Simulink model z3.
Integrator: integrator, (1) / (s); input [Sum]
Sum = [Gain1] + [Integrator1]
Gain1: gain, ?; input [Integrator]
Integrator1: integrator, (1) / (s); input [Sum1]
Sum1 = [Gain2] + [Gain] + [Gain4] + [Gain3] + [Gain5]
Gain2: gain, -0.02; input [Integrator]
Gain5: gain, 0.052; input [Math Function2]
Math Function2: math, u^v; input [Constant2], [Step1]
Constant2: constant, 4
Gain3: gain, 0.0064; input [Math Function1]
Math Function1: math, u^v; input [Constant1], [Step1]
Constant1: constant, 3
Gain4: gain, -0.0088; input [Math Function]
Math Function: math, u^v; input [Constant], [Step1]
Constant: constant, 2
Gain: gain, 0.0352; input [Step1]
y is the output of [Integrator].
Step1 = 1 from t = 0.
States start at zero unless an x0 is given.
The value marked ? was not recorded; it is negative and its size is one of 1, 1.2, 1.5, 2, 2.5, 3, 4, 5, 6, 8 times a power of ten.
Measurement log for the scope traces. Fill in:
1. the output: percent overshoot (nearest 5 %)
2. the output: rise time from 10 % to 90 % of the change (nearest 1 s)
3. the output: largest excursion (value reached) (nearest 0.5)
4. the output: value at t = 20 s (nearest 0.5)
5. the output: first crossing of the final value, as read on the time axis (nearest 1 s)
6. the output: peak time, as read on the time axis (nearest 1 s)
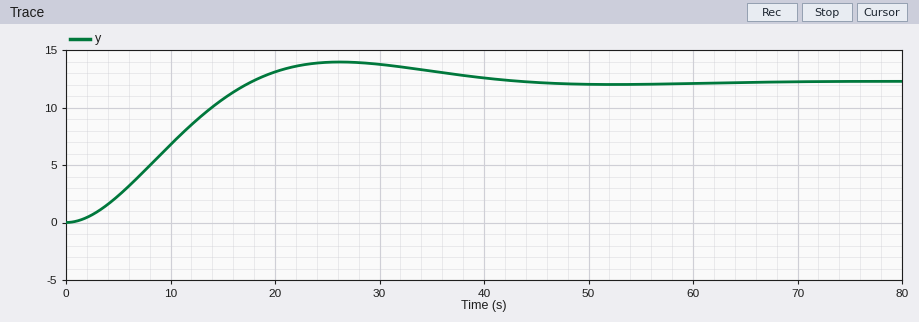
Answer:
15 %
12 s
14.0
13.0
18 s
26 s
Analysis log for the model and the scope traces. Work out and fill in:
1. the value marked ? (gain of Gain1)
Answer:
-0.15
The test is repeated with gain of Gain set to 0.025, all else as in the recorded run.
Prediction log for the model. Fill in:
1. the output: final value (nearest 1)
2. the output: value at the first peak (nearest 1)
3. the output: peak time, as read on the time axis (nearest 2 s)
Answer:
12
13
26 s
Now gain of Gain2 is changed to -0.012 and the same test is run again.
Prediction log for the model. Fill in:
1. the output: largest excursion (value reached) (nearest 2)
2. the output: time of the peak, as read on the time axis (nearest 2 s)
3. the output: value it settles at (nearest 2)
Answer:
22
40 s
20
